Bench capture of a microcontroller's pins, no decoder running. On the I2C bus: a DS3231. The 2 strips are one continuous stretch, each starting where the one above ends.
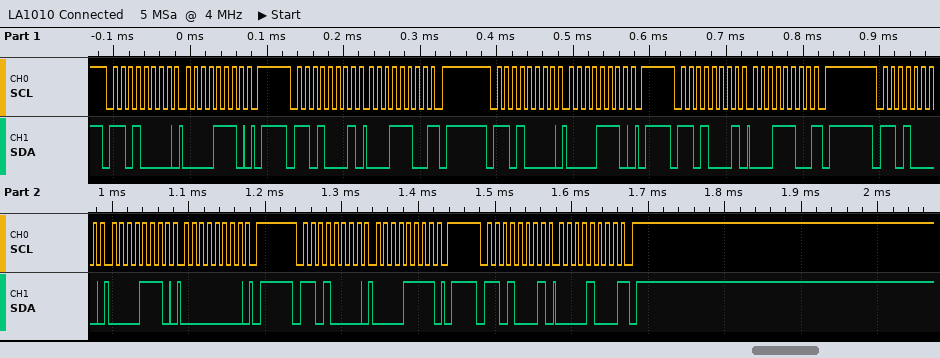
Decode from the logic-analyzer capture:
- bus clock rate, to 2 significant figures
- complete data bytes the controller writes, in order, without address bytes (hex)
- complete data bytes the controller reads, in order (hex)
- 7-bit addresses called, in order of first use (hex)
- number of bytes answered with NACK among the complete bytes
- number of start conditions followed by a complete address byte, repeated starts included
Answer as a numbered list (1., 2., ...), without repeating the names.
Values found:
1. 100 kHz
2. 0E 0E 0E 00 0F
3. 1C 1C 08
4. 0x68
5. 3
6. 7
